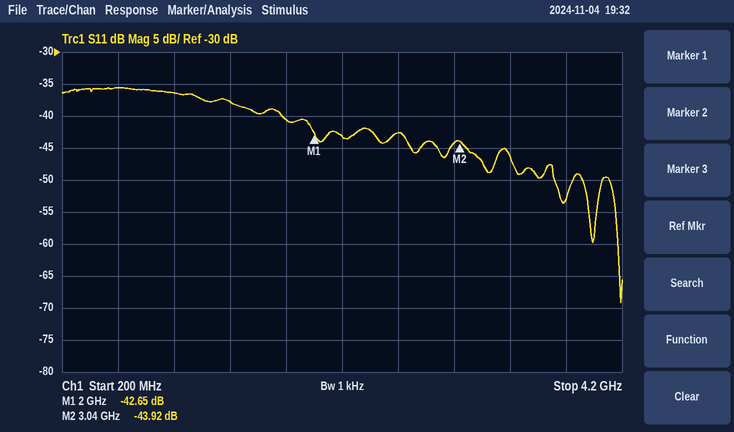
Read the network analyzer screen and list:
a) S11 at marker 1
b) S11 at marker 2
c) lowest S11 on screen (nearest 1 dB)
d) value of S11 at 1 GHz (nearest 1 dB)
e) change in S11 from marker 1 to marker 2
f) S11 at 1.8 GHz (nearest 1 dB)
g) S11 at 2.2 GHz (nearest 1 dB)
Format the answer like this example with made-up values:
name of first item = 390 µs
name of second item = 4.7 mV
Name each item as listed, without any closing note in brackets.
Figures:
S11 at marker 1 = -42.65 dB
S11 at marker 2 = -43.92 dB
lowest S11 on screen = -69 dB
value of S11 at 1 GHz = -36 dB
change in S11 from marker 1 to marker 2 = -1.27 dB
S11 at 1.8 GHz = -41 dB
S11 at 2.2 GHz = -43 dB
